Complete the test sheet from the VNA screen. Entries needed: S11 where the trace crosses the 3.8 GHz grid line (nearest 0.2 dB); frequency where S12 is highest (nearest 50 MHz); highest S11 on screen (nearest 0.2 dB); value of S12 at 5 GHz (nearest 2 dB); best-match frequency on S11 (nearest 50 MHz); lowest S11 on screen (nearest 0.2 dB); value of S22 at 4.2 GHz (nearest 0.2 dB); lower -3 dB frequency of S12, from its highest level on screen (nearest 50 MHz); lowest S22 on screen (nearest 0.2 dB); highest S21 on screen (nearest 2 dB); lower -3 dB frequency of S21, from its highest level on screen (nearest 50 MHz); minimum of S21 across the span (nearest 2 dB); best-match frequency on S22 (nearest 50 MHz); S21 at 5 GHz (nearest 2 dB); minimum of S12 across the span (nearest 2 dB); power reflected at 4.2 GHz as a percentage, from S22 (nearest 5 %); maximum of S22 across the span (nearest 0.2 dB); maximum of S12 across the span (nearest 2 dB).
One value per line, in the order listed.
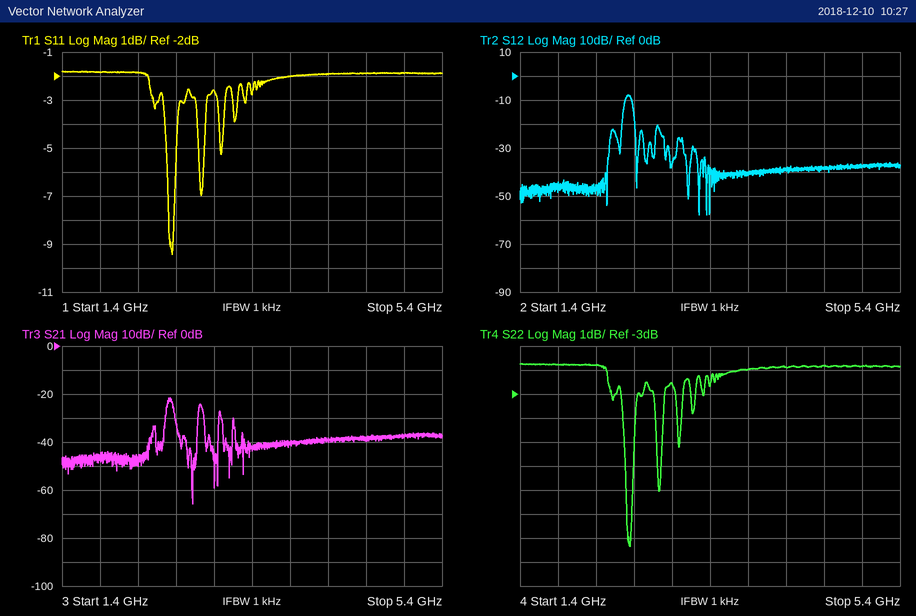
-2.0 dB
2.55 GHz
-1.8 dB
-38 dB
2.55 GHz
-9.4 dB
-1.8 dB
2.50 GHz
-9.4 dB
-22 dB
2.50 GHz
-66 dB
2.55 GHz
-38 dB
-58 dB
65 %
-1.8 dB
-8 dB
